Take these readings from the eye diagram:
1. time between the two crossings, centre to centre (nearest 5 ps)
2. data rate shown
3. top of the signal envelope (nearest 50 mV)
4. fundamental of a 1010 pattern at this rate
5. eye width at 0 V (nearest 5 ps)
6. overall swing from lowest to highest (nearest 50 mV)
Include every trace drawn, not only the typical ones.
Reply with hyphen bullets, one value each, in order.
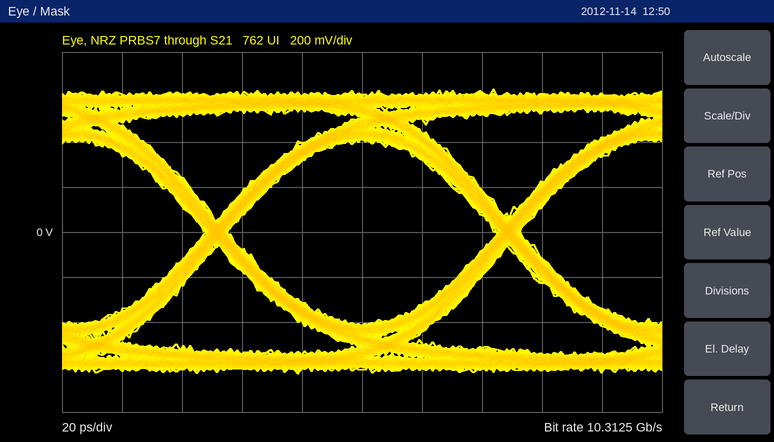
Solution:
- 95 ps
- 10.3125 Gb/s
- 650 mV
- 5.15625 GHz
- 90 ps
- 1.25 V
